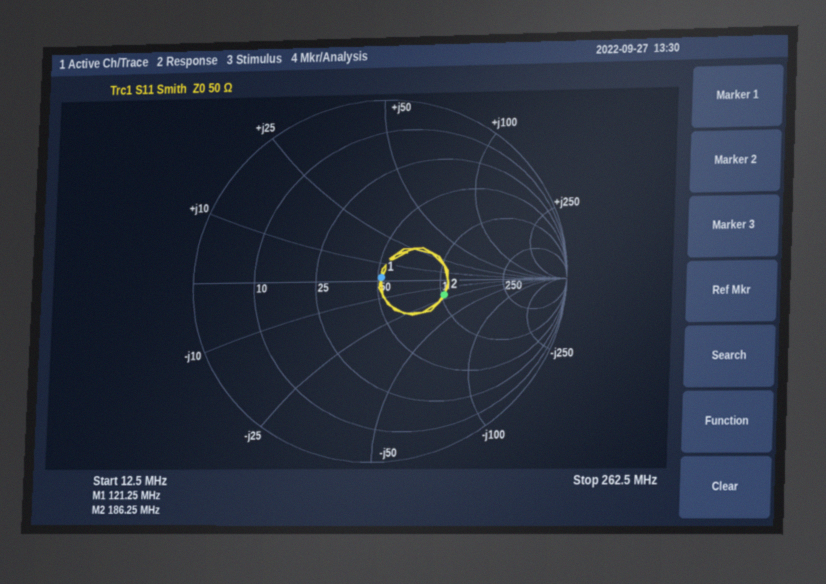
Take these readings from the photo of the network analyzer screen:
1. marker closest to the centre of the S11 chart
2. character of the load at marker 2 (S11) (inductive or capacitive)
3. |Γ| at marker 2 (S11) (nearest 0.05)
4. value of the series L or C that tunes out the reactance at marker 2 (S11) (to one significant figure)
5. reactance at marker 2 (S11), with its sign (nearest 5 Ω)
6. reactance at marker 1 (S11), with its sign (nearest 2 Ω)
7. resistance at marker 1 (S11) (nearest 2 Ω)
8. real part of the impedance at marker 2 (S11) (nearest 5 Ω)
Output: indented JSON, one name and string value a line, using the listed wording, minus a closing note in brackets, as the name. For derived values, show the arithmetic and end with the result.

{
  "marker closest to the centre of the S11 chart": "marker 1",
  "character of the load at marker 2 (S11)": "capacitive",
  "|Γ| at marker 2 (S11)": "0.35",
  "value of the series L or C that tunes out the reactance at marker 2 (S11)": "L = 20 Ω/(2π × 186.25 MHz) ≈ 17.1 nH, so 20 nH to one significant figure",
  "reactance at marker 2 (S11), with its sign": "-20 Ω",
  "reactance at marker 1 (S11), with its sign": "+2 Ω",
  "resistance at marker 1 (S11)": "52 Ω",
  "real part of the impedance at marker 2 (S11)": "105 Ω"
}
